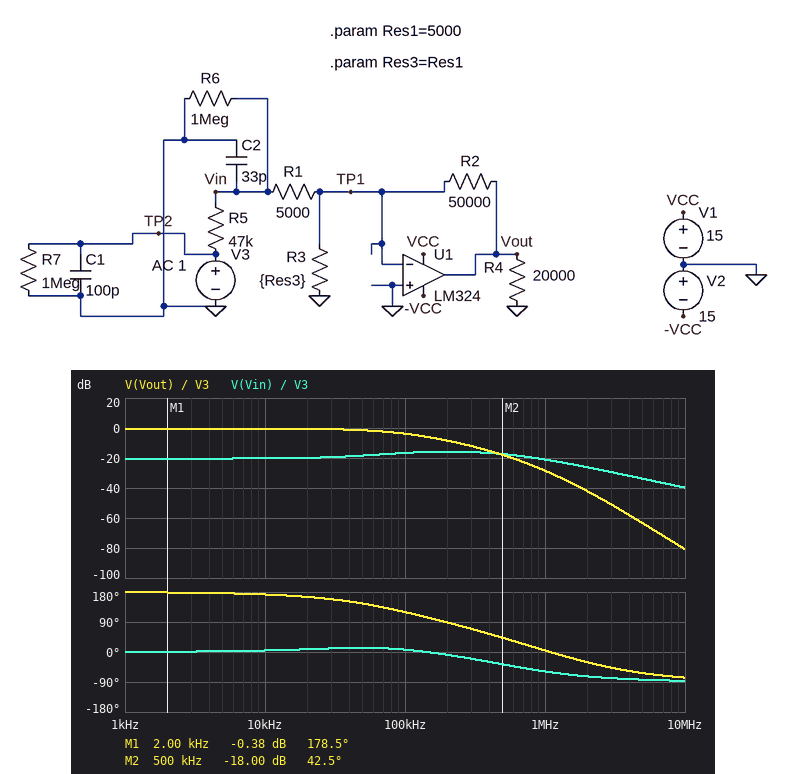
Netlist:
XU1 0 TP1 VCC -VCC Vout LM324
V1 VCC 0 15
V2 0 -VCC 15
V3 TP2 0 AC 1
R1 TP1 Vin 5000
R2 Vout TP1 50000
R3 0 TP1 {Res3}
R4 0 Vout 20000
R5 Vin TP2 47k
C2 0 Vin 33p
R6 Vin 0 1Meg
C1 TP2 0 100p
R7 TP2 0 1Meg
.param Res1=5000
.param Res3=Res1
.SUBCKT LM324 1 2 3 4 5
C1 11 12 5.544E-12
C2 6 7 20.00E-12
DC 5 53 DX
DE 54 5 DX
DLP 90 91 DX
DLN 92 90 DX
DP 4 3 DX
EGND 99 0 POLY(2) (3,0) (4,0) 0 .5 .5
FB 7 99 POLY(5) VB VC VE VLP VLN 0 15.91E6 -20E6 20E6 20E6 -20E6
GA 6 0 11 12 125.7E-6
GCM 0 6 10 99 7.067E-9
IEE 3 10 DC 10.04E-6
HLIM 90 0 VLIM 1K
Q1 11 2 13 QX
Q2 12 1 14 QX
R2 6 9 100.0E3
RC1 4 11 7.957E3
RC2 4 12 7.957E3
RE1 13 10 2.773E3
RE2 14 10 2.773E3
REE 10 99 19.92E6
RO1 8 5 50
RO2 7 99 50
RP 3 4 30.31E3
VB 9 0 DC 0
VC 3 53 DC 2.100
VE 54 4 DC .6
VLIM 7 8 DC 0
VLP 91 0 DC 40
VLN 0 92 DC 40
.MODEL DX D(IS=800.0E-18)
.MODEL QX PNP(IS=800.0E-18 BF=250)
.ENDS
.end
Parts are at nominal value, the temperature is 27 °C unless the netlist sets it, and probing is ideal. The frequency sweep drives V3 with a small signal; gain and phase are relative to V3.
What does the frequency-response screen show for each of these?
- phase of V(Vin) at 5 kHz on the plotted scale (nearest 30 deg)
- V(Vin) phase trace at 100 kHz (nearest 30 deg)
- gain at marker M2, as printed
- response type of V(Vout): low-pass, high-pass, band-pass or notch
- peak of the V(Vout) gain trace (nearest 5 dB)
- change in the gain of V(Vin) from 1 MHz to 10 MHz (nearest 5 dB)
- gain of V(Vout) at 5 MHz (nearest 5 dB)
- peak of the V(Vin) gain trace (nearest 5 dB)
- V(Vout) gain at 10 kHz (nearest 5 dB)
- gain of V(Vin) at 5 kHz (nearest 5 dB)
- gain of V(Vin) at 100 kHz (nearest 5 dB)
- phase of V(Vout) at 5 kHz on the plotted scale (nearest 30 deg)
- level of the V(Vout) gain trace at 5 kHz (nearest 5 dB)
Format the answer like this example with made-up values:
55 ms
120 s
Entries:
0 deg
0 deg
-18.00 dB
low-pass
0 dB
-20 dB
-65 dB
-15 dB
0 dB
-20 dB
-15 dB
180 deg
0 dB
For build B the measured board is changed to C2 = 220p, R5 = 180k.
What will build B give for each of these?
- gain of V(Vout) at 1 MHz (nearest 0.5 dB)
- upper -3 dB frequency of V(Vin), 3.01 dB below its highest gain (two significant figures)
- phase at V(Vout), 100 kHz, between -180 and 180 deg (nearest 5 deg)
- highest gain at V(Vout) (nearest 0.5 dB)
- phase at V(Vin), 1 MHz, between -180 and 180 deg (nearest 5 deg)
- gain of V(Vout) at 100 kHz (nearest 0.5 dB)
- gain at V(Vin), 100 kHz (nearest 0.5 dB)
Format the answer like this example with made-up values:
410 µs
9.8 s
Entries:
-55.5 dB
150 kHz
75 deg
-11.5 dB
-85 deg
-16.5 dB
-29.5 dB
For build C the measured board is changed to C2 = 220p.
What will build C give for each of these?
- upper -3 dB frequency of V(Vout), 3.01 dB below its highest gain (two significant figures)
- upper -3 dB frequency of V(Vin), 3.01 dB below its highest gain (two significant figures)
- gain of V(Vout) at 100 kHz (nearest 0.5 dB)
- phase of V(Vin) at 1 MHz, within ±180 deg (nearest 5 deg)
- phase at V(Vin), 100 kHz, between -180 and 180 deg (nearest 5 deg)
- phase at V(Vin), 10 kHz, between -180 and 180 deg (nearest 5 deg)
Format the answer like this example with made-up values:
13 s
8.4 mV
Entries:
79 kHz
160 kHz
-5.5 dB
-85 deg
-35 deg
0 deg
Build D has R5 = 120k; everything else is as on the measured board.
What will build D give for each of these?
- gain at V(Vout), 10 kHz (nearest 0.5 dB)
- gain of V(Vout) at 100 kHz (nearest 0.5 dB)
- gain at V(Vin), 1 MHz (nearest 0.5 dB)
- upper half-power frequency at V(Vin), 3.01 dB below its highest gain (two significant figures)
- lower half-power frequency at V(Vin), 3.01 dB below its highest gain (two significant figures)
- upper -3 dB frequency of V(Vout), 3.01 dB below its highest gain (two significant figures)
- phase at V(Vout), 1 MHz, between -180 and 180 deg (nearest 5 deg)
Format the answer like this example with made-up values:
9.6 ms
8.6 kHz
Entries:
-8.0 dB
-11.0 dB
-29.0 dB
630 kHz
46 kHz
97 kHz
0 deg
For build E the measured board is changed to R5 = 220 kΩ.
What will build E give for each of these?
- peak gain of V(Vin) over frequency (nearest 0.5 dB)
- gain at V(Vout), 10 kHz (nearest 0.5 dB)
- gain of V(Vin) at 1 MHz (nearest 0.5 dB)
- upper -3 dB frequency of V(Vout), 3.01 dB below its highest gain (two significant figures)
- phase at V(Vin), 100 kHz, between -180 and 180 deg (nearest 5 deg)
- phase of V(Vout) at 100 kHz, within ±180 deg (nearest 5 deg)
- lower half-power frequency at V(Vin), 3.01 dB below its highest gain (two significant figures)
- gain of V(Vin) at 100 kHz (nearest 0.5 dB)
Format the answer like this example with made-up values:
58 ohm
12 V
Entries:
-28.0 dB
-13.0 dB
-34.0 dB
99 kHz
10 deg
120 deg
48 kHz
-29.0 dB
